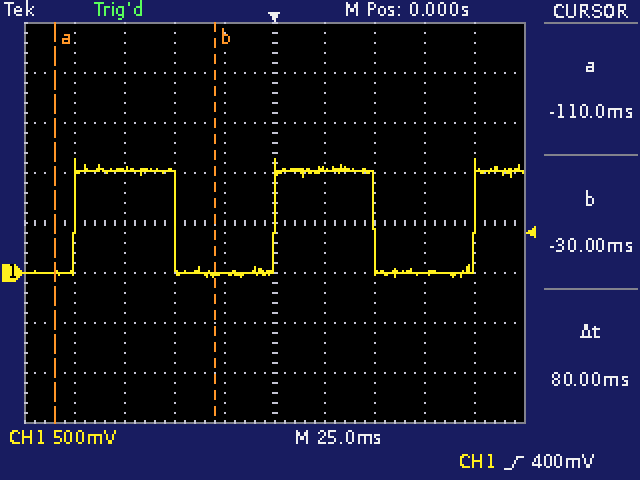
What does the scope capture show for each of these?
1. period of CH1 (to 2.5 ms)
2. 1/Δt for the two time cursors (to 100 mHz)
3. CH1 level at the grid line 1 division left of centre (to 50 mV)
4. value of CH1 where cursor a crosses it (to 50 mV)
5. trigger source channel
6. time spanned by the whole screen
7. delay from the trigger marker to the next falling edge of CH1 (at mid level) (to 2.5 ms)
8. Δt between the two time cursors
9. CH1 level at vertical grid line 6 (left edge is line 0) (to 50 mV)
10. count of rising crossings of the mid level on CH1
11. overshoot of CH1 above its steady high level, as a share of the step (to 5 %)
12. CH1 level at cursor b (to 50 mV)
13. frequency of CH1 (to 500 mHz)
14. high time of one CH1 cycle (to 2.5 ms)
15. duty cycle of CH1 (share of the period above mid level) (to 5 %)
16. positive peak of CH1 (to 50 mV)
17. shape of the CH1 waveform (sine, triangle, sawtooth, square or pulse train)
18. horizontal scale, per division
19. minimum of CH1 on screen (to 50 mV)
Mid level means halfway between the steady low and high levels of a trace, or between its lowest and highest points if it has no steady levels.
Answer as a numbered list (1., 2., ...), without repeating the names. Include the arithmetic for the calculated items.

1. 100.0 ms
2. 1 / 80 ms ≈ 12.5 Hz
3. 0 mV
4. 0 mV
5. CH1
6. 250 ms
7. 50.0 ms
8. 80 ms
9. 1.05 V
10. 3
11. 10 %
12. 0 mV
13. 1 / 100.0 ms ≈ 10.0 Hz
14. 50.0 ms
15. 50.0 ms / 100.0 ms ≈ 50 %
16. 1.15 V
17. square
18. 25 ms
19. -50 mV
